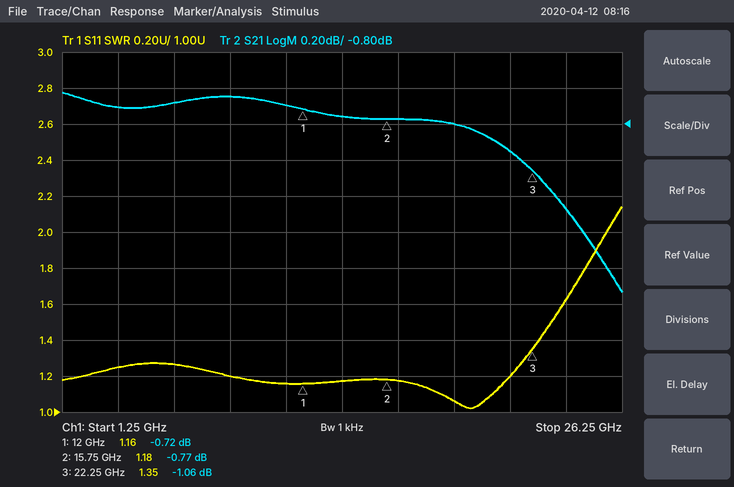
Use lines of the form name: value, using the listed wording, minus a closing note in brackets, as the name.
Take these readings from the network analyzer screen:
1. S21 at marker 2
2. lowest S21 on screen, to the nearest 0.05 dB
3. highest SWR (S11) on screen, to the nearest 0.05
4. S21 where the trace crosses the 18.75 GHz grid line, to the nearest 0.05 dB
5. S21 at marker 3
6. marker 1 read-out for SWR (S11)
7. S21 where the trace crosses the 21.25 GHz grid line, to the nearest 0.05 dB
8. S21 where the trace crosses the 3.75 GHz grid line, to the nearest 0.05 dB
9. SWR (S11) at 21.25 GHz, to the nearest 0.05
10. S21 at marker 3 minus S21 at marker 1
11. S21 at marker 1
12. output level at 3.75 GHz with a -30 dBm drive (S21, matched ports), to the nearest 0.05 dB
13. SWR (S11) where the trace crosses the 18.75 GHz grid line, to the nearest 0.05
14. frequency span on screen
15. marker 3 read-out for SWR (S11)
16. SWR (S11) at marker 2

S21 at marker 2: -0.77 dB
lowest S21 on screen, to the nearest 0.05 dB: -1.75 dB
highest SWR (S11) on screen, to the nearest 0.05: 2.15
S21 where the trace crosses the 18.75 GHz grid line, to the nearest 0.05 dB: -0.80 dB
S21 at marker 3: -1.06 dB
marker 1 read-out for SWR: 1.16
S21 where the trace crosses the 21.25 GHz grid line, to the nearest 0.05 dB: -0.95 dB
S21 where the trace crosses the 3.75 GHz grid line, to the nearest 0.05 dB: -0.70 dB
SWR (S11) at 21.25 GHz, to the nearest 0.05: 1.20
S21 at marker 3 minus S21 at marker 1: -0.34 dB
S21 at marker 1: -0.72 dB
output level at 3.75 GHz with a -30 dBm drive (S21, matched ports), to the nearest 0.05 dB: -30.70 dBm
SWR (S11) where the trace crosses the 18.75 GHz grid line, to the nearest 0.05: 1.05
frequency span on screen: 25 GHz
marker 3 read-out for SWR: 1.35
SWR (S11) at marker 2: 1.18
